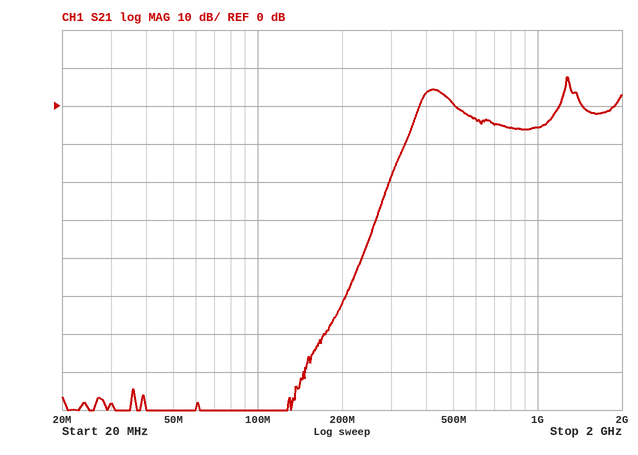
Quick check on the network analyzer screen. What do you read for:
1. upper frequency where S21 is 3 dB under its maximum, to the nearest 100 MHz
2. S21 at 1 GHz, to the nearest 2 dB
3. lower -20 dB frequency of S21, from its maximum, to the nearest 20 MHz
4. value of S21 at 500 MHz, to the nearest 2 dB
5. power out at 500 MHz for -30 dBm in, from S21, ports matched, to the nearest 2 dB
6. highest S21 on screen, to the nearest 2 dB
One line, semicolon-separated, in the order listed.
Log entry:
1.3 GHz; -6 dB; 320 MHz; 0 dB; -30 dBm; 8 dB
